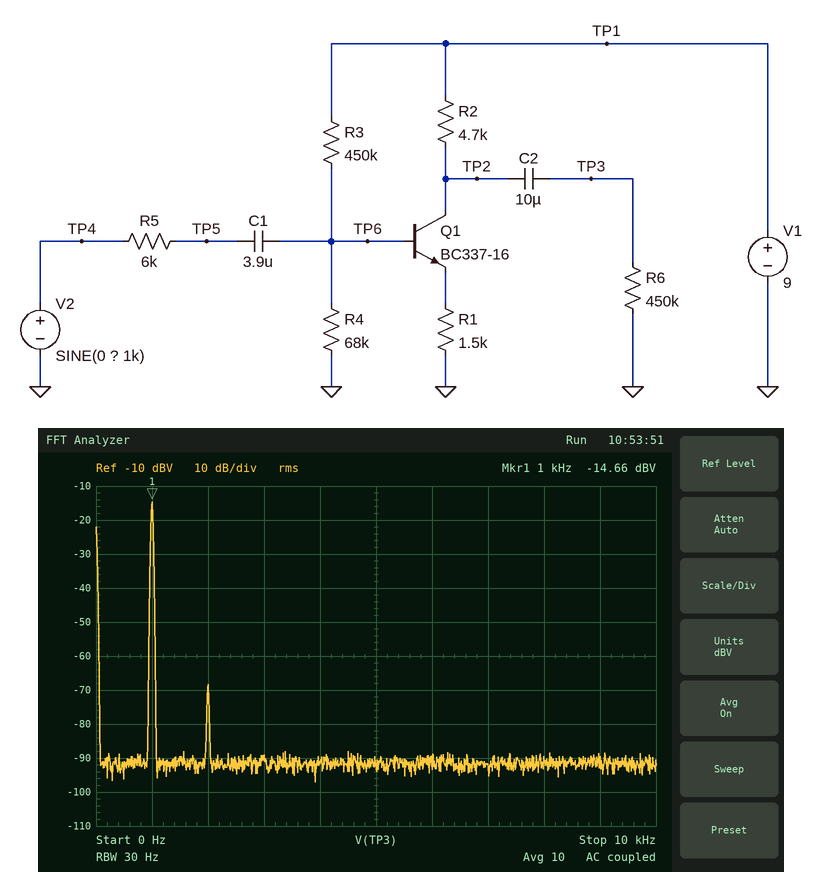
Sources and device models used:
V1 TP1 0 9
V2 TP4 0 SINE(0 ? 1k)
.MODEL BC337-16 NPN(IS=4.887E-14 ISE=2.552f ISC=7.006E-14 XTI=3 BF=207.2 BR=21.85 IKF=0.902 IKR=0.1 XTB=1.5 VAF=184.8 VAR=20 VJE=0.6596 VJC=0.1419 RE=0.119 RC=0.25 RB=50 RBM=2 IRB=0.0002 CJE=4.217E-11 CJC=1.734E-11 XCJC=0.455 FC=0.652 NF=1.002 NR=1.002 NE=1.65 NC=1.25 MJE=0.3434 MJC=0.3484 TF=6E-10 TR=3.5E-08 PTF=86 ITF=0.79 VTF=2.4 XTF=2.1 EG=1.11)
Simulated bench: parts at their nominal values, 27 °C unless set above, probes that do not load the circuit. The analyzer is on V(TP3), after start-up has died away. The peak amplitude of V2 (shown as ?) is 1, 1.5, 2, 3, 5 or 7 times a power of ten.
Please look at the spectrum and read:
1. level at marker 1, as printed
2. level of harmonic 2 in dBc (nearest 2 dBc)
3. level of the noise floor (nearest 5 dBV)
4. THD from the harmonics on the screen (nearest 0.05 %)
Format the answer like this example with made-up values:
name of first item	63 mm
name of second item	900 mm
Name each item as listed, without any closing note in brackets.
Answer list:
level at marker 1, as printed	-14.66 dBV
level of harmonic 2 in dBc	-54 dBc
level of the noise floor	-90 dBV
THD from the harmonics on the screen	0.20 %
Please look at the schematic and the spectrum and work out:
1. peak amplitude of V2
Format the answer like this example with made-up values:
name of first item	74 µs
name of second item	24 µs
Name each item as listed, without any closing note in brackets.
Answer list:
peak amplitude of V2	100 mV
